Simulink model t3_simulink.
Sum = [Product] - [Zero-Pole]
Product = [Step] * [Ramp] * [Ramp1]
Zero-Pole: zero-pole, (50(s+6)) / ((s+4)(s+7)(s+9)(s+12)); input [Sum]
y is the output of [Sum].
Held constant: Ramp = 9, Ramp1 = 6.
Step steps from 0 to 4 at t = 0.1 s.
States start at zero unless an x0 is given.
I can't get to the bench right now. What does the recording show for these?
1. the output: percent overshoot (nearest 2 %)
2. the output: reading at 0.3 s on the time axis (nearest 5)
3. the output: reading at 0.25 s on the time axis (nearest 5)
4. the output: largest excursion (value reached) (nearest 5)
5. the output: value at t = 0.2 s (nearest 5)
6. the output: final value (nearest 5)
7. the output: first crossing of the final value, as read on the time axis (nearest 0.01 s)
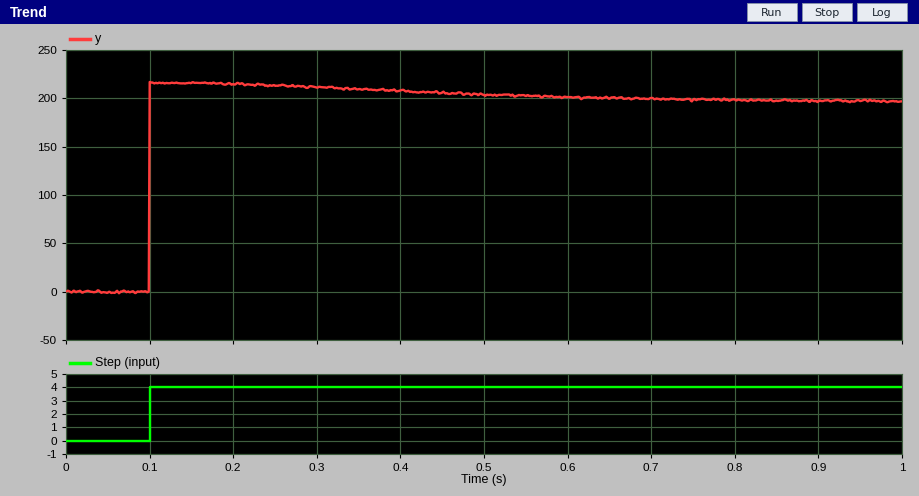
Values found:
10 %
210
215
215
215
195
0.10 s
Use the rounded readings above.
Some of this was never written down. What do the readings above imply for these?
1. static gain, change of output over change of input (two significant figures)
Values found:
49
